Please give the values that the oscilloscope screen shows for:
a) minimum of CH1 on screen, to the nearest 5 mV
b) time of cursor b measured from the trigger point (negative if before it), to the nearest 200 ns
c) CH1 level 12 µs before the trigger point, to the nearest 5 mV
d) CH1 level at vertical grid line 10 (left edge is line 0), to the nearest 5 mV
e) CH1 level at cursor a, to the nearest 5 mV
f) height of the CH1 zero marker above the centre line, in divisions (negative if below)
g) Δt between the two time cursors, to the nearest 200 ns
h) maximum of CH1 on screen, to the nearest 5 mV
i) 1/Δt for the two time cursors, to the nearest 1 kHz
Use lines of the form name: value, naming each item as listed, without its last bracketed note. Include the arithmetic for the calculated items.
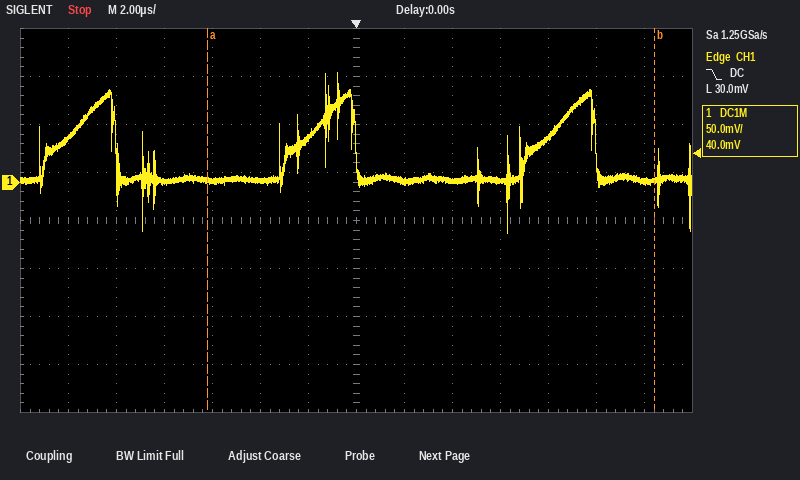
minimum of CH1 on screen, to the nearest 5 mV: -55 mV
time of cursor b measured from the trigger point (negative if before it), to the nearest 200 ns: +12.4 µs
CH1 level 12 µs before the trigger point, to the nearest 5 mV: 45 mV
CH1 level at vertical grid line 10 (left edge is line 0), to the nearest 5 mV: 0 mV
CH1 level at cursor a, to the nearest 5 mV: 0 mV
height of the CH1 zero marker above the centre line, in divisions: +0.8 div
Δt between the two time cursors, to the nearest 200 ns: 18.6 µs
maximum of CH1 on screen, to the nearest 5 mV: 115 mV
1/Δt for the two time cursors, to the nearest 1 kHz: 1 / 18.6 µs ≈ 54 kHz
